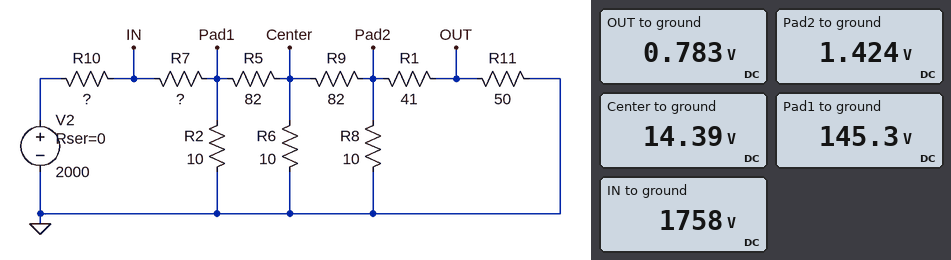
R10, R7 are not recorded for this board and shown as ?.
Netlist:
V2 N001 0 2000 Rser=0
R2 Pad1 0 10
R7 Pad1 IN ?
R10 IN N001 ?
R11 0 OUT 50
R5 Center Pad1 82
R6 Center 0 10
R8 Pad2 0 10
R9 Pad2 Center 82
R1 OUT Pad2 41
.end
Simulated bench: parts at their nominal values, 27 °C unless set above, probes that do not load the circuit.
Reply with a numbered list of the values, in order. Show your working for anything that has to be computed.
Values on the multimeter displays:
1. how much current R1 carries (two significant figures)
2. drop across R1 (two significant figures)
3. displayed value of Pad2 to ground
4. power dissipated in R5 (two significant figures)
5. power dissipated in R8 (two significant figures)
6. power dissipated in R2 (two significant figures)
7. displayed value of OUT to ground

1. (1.424 V - 783 mV) / 41 Ω = 16 mA
2. 1.424 V - 783 mV = 640 mV
3. 1.424 V
4. (145.3 V - 14.39 V)^2 / 82 Ω = 210 W
5. (1.424 V)^2 / 10 Ω = 200 mW
6. (145.3 V)^2 / 10 Ω = 2.1 kW
7. 0.783 V
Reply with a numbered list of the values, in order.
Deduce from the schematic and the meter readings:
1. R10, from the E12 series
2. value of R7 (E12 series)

1. 15 Ω
2. 100 Ω
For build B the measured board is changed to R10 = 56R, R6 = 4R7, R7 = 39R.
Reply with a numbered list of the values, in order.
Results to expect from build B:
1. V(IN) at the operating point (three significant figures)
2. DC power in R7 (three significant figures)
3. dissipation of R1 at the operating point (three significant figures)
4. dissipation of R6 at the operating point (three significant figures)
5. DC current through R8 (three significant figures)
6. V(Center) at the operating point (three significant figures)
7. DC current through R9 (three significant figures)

1. 923 V
2. 14.4 kW
3. 3.85 mW
4. 16.9 W
5. 88.2 mA
6. 8.91 V
7. 97.9 mA
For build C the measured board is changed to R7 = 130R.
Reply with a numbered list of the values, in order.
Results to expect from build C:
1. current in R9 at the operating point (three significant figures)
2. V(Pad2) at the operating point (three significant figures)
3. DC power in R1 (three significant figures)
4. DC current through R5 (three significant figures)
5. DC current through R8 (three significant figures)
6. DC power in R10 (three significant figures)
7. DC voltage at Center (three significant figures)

1. 127 mA
2. 1.15 V
3. 6.51 mW
4. 1.29 A
5. 115 mA
6. 2.53 kW
7. 11.6 V
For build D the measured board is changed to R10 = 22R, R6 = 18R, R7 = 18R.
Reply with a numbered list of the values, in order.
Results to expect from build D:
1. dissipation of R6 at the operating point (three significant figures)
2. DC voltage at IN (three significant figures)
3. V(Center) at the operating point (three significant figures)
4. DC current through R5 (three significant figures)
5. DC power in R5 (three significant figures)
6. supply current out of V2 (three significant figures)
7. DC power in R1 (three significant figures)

1. 182 W
2. 1.10 kV
3. 57.2 V
4. 3.81 A
5. 1.19 kW
6. 40.8 A
7. 159 mW
